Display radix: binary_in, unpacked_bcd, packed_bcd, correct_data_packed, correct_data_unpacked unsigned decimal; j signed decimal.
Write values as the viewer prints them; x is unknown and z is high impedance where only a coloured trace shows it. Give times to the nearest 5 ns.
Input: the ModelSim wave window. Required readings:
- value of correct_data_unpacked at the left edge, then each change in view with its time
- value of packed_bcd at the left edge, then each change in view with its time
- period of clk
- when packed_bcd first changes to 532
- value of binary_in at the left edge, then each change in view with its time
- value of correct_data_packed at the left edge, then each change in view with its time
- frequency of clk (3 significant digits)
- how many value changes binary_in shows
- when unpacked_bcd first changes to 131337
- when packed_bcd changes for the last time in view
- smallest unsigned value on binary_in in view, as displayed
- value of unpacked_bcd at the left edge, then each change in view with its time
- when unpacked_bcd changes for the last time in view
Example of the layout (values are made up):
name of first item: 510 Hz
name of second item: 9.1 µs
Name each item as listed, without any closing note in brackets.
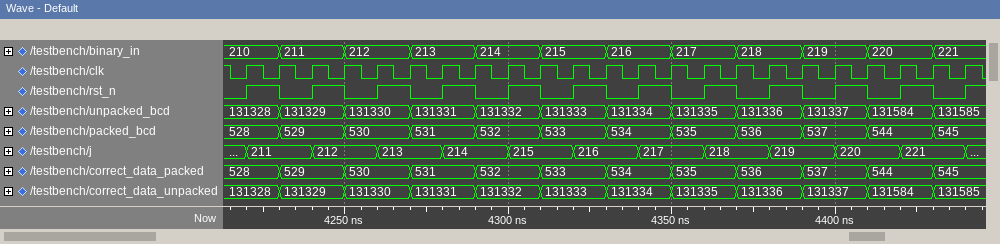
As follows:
value of correct_data_unpacked at the left edge, then each change in view with its time: 131328, 131329 at 4230 ns, 131330 at 4250 ns, 131331 at 4270 ns, 131332 at 4290 ns, 131333 at 4310 ns, 131334 at 4330 ns, 131335 at 4350 ns, 131336 at 4370 ns, 131337 at 4390 ns, 131584 at 4410 ns, 131585 at 4430 ns
value of packed_bcd at the left edge, then each change in view with its time: 528, 529 at 4230 ns, 530 at 4250 ns, 531 at 4270 ns, 532 at 4290 ns, 533 at 4310 ns, 534 at 4330 ns, 535 at 4350 ns, 536 at 4370 ns, 537 at 4390 ns, 544 at 4410 ns, 545 at 4430 ns
period of clk: 10 ns
when packed_bcd first changes to 532: 4290 ns
value of binary_in at the left edge, then each change in view with its time: 210, 211 at 4230 ns, 212 at 4250 ns, 213 at 4270 ns, 214 at 4290 ns, 215 at 4310 ns, 216 at 4330 ns, 217 at 4350 ns, 218 at 4370 ns, 219 at 4390 ns, 220 at 4410 ns, 221 at 4430 ns
value of correct_data_packed at the left edge, then each change in view with its time: 528, 529 at 4230 ns, 530 at 4250 ns, 531 at 4270 ns, 532 at 4290 ns, 533 at 4310 ns, 534 at 4330 ns, 535 at 4350 ns, 536 at 4370 ns, 537 at 4390 ns, 544 at 4410 ns, 545 at 4430 ns
frequency of clk: 100 MHz
how many value changes binary_in shows: 11
when unpacked_bcd first changes to 131337: 4390 ns
when packed_bcd changes for the last time in view: 4430 ns
smallest unsigned value on binary_in in view, as displayed: 210
value of unpacked_bcd at the left edge, then each change in view with its time: 131328, 131329 at 4230 ns, 131330 at 4250 ns, 131331 at 4270 ns, 131332 at 4290 ns, 131333 at 4310 ns, 131334 at 4330 ns, 131335 at 4350 ns, 131336 at 4370 ns, 131337 at 4390 ns, 131584 at 4410 ns, 131585 at 4430 ns
when unpacked_bcd changes for the last time in view: 4430 ns
